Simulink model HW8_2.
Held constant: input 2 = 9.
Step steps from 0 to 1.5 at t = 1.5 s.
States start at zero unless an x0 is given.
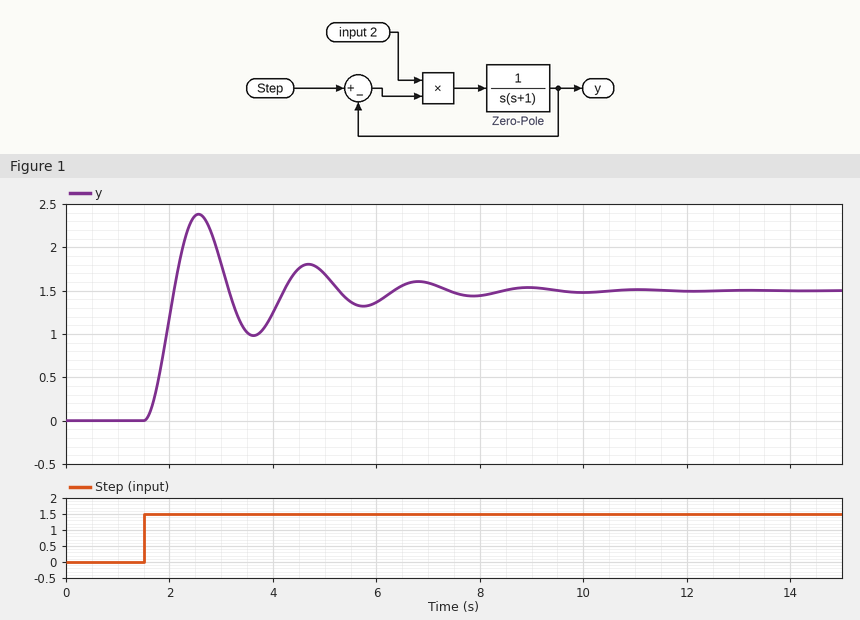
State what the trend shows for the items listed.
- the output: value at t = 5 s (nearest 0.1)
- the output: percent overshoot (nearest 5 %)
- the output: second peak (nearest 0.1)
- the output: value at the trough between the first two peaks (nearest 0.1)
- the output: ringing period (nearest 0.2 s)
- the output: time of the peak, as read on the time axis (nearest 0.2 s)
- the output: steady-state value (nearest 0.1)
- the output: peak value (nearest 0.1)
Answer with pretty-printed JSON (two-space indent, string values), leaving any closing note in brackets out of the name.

{
  "the output: value at t = 5 s": "1.7",
  "the output: percent overshoot": "60 %",
  "the output: second peak": "1.8",
  "the output: value at the trough between the first two peaks": "1.0",
  "the output: ringing period": "2.2 s",
  "the output: time of the peak, as read on the time axis": "2.6 s",
  "the output: steady-state value": "1.5",
  "the output: peak value": "2.4"
}
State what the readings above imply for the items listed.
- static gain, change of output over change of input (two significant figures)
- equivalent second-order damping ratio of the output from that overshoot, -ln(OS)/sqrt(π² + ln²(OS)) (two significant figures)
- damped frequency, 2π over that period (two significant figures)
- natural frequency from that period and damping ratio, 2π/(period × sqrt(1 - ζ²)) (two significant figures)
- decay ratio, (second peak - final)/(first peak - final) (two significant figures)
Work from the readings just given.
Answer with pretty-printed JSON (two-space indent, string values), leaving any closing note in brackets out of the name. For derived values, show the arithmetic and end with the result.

{
  "static gain, change of output over change of input": "(1.5 - 0) / (1.5 - 0) = 1.0",
  "equivalent second-order damping ratio of the output from that overshoot, -ln(OS)/sqrt(π² + ln²(OS))": "ln(0.6) = -0.511; 0.511 / sqrt(9.870 + 0.261) = 0.16",
  "damped frequency, 2π over that period": "2π / 2.2 = 2.9 rad/s",
  "natural frequency from that period and damping ratio, 2π/(period × sqrt(1 - ζ²))": "2π / (2.2 × sqrt(1 - 0.16²)) = 2.9 rad/s",
  "decay ratio, (second peak - final)/(first peak - final)": "(1.8 - 1.5) / (2.4 - 1.5) = 0.33"
}
